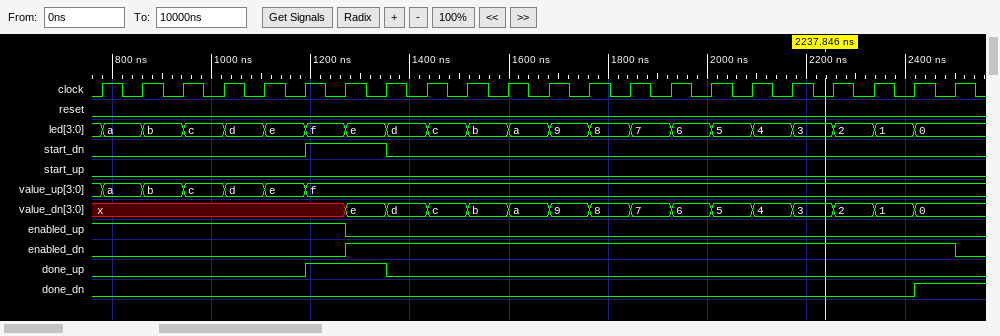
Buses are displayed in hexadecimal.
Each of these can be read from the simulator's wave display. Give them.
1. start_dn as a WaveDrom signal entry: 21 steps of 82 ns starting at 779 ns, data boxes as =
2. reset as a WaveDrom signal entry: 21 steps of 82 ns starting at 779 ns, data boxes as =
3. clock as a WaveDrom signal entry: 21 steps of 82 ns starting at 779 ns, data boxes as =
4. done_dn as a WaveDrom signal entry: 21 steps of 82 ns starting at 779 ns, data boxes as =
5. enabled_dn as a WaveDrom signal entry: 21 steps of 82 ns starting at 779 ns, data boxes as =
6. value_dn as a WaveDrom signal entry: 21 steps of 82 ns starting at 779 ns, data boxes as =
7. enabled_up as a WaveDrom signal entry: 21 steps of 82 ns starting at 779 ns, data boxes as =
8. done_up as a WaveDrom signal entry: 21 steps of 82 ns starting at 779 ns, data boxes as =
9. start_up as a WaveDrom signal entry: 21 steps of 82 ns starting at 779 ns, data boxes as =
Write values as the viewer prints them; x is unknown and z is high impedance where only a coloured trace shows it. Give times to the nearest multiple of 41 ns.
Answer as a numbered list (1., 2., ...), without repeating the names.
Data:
1. {name: 'start_dn', wave: '0....1.0.............'}
2. {name: 'reset', wave: '0....................'}
3. {name: 'clock', wave: 'p....................'}
4. {name: 'done_dn', wave: '0...................1'}
5. {name: 'enabled_dn', wave: '0.....1..............'}
6. {name: 'value_dn', wave: 'x.....===============', data: 'e d c b a 9 8 7 6 5 4 3 2 1 0'}
7. {name: 'enabled_up', wave: '1.....0..............'}
8. {name: 'done_up', wave: '0....1.0.............'}
9. {name: 'start_up', wave: '0....................'}
